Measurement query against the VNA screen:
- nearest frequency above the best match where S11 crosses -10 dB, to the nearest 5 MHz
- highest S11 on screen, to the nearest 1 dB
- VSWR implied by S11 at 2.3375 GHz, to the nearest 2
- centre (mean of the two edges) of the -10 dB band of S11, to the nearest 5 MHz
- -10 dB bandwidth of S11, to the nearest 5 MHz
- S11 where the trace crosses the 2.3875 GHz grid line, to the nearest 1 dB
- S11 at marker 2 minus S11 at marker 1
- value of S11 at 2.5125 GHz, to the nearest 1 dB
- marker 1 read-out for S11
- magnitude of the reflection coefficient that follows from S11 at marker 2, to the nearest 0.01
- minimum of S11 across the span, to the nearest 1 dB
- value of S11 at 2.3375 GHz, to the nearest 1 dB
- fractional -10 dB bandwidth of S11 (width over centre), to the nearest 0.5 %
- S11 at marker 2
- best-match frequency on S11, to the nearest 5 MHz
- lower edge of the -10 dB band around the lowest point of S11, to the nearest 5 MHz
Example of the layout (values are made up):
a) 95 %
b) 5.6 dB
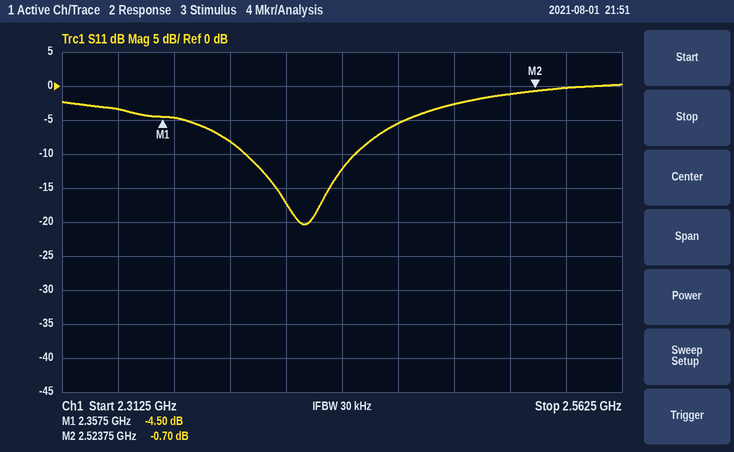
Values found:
a) 2.445 GHz
b) 0 dB
c) 6
d) 2.420 GHz
e) 50 MHz
f) -8 dB
g) 3.80 dB
h) -1 dB
i) -4.50 dB
j) 0.92
k) -20 dB
l) -3 dB
m) 2.0 %
n) -0.70 dB
o) 2.420 GHz
p) 2.395 GHz
